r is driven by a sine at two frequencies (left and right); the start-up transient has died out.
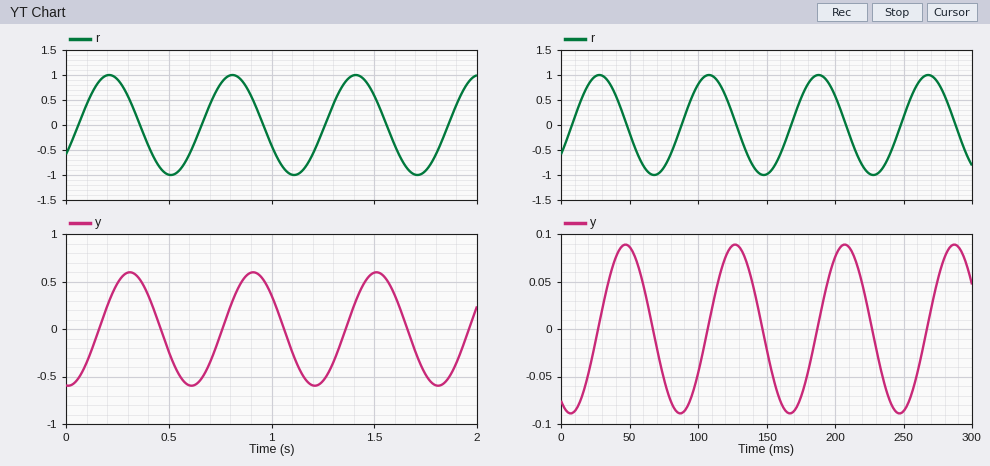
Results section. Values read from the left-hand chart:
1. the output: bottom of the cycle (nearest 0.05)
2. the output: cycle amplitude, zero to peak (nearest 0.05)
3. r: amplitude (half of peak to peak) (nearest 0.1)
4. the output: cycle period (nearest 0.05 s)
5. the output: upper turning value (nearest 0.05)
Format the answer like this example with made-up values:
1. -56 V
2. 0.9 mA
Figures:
1. -0.60
2. 0.60
3. 1.0
4. 0.60 s
5. 0.60
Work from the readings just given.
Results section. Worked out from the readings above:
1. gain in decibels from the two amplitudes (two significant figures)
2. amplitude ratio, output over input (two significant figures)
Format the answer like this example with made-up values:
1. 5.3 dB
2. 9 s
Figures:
1. -4.4 dB
2. 0.60
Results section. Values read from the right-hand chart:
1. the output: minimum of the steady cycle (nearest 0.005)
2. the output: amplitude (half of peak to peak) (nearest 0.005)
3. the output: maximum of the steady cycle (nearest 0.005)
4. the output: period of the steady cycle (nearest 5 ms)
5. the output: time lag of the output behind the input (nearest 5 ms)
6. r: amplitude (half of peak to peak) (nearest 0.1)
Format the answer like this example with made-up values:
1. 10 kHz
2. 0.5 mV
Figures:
1. -0.090
2. 0.090
3. 0.090
4. 80 ms
5. 20 ms
6. 1.0
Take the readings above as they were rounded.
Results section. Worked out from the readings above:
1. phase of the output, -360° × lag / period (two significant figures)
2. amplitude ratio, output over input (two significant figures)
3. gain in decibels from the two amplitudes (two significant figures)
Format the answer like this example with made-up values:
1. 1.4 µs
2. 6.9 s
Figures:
1. -90°
2. 0.090
3. -21 dB
